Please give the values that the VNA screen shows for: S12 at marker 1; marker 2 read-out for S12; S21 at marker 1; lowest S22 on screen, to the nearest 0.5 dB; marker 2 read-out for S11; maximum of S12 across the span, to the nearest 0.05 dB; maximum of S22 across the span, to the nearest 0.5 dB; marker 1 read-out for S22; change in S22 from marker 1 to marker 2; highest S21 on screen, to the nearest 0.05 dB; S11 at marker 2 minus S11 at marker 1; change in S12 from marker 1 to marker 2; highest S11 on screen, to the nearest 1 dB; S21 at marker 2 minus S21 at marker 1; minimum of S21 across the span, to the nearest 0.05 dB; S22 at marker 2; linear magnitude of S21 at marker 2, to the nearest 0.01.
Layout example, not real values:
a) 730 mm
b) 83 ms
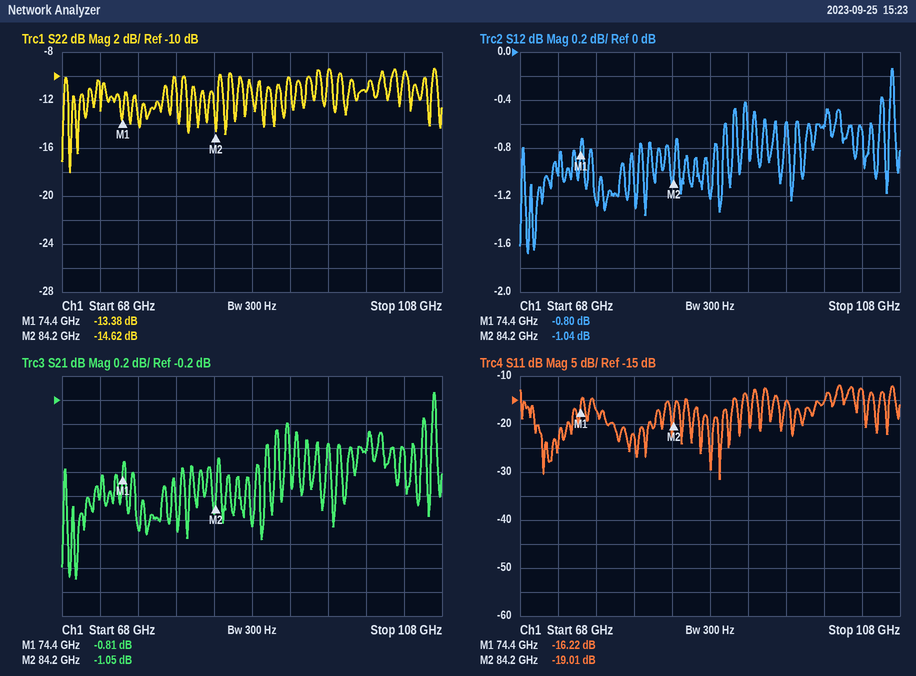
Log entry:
a) -0.80 dB
b) -1.04 dB
c) -0.81 dB
d) -18.0 dB
e) -19.01 dB
f) -0.15 dB
g) -9.5 dB
h) -13.38 dB
i) -1.24 dB
j) -0.15 dB
k) -2.79 dB
l) -0.24 dB
m) -12 dB
n) -0.24 dB
o) -1.70 dB
p) -14.62 dB
q) 0.89
